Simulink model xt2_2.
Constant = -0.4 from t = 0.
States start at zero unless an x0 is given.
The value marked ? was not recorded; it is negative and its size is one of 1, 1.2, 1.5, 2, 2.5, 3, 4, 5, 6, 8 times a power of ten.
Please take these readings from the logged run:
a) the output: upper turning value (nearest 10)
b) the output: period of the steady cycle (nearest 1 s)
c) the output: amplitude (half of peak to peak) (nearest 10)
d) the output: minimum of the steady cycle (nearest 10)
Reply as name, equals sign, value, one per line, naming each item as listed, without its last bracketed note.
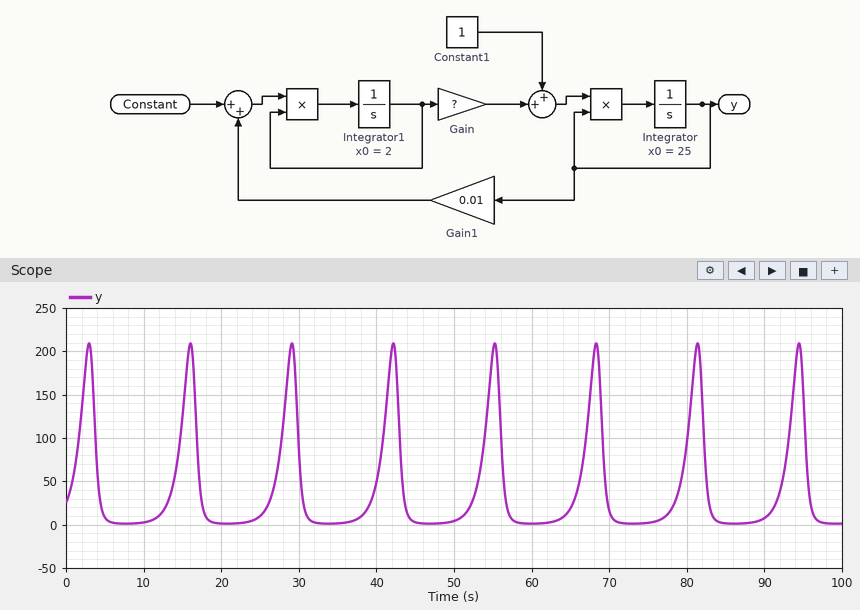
the output: upper turning value = 210
the output: period of the steady cycle = 13 s
the output: amplitude (half of peak to peak) = 100
the output: minimum of the steady cycle = 0
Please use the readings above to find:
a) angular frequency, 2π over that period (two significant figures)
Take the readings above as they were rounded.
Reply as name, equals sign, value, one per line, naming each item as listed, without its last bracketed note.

angular frequency, 2π over that period = 0.48 rad/s
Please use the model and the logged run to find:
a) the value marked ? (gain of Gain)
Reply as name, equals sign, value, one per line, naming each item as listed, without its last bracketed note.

the value marked ? = -0.08
